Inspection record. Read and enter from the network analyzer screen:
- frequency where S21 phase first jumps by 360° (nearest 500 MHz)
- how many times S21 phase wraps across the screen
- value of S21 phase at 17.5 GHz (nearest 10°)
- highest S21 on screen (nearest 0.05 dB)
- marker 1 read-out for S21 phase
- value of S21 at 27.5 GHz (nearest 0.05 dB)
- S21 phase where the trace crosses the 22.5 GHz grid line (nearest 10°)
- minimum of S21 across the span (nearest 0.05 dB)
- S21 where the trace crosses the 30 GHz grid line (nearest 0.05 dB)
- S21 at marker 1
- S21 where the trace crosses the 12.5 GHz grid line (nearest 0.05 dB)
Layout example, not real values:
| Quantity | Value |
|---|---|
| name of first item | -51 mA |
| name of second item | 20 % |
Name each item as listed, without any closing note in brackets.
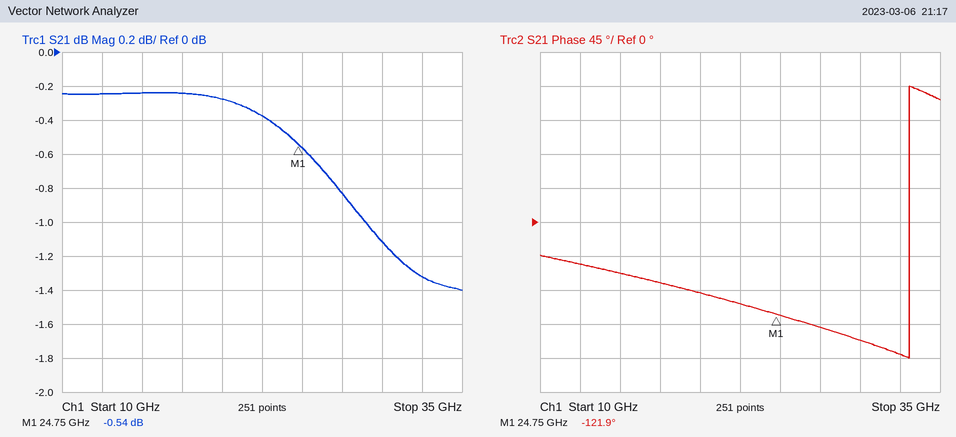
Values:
| Quantity | Value |
|---|---|
| frequency where S21 phase first jumps by 360° | 33.0 GHz |
| how many times S21 phase wraps across the screen | 1 |
| value of S21 phase at 17.5 GHz | -80° |
| highest S21 on screen | -0.25 dB |
| marker 1 read-out for S21 phase | -121.9° |
| value of S21 at 27.5 GHz | -0.85 dB |
| S21 phase where the trace crosses the 22.5 GHz grid line | -110° |
| minimum of S21 across the span | -1.40 dB |
| S21 where the trace crosses the 30 GHz grid line | -1.10 dB |
| S21 at marker 1 | -0.54 dB |
| S21 where the trace crosses the 12.5 GHz grid line | -0.25 dB |
